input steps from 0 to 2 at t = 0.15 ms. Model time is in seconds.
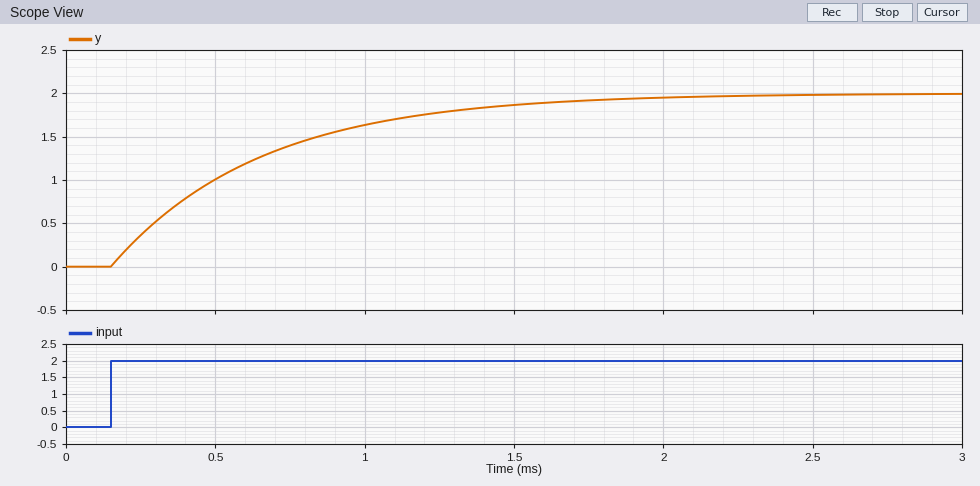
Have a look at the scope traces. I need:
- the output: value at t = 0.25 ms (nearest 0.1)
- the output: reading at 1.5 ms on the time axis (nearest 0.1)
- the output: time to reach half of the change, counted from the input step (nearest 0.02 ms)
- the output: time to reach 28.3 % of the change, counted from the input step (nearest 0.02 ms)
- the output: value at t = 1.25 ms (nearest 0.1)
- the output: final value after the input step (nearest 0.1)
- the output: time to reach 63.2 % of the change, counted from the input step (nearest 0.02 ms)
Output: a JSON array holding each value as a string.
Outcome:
["0.4", "1.9", "0.34 ms", "0.16 ms", "1.8", "2.0", "0.50 ms"]
